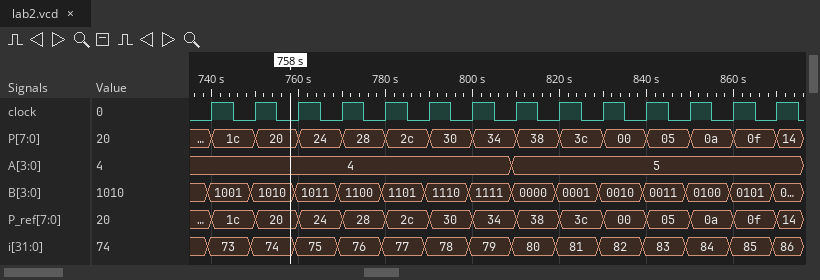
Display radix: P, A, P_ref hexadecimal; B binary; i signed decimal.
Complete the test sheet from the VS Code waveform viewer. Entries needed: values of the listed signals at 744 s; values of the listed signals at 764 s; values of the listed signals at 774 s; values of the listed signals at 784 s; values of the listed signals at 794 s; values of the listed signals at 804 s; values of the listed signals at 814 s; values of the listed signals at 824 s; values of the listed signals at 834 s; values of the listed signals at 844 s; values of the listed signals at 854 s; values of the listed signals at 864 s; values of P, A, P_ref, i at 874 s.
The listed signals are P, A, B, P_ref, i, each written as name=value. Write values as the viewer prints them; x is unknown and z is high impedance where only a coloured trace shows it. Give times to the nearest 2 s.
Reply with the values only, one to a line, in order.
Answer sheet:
P=1c, A=4, B=1001, P_ref=1c, i=73
P=24, A=4, B=1011, P_ref=24, i=75
P=28, A=4, B=1100, P_ref=28, i=76
P=2c, A=4, B=1101, P_ref=2c, i=77
P=30, A=4, B=1110, P_ref=30, i=78
P=34, A=4, B=1111, P_ref=34, i=79
P=38, A=5, B=0000, P_ref=38, i=80
P=3c, A=5, B=0001, P_ref=3c, i=81
P=00, A=5, B=0010, P_ref=00, i=82
P=05, A=5, B=0011, P_ref=05, i=83
P=0a, A=5, B=0100, P_ref=0a, i=84
P=0f, A=5, B=0101, P_ref=0f, i=85
P=14, A=5, P_ref=14, i=86
